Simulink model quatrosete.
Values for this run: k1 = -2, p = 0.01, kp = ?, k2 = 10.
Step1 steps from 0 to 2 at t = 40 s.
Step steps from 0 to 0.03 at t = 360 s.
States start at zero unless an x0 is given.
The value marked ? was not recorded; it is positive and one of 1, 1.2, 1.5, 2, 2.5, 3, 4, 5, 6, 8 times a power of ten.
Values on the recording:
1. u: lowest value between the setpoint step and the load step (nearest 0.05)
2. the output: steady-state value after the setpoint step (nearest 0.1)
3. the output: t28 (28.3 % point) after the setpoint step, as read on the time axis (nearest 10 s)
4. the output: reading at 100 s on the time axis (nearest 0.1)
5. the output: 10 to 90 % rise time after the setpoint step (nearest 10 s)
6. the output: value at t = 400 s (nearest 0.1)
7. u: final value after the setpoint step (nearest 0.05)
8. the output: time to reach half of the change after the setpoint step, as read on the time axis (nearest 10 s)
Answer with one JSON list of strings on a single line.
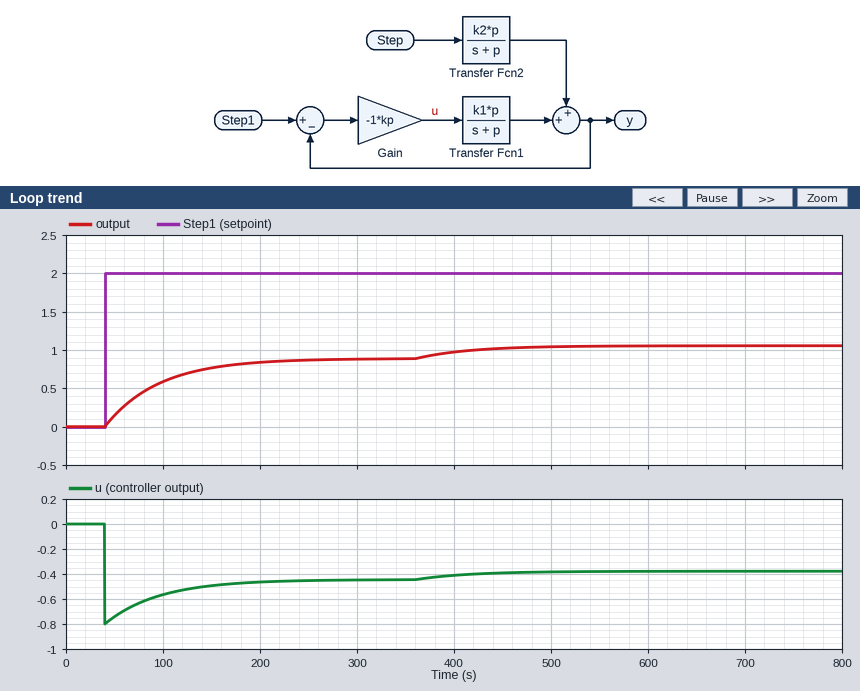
["-0.80", "0.9", "60 s", "0.6", "120 s", "1.0", "-0.45", "80 s"]
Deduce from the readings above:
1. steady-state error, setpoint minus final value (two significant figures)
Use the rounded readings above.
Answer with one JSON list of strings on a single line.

["1.1"]
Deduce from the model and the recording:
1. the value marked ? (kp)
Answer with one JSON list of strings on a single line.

["0.4"]
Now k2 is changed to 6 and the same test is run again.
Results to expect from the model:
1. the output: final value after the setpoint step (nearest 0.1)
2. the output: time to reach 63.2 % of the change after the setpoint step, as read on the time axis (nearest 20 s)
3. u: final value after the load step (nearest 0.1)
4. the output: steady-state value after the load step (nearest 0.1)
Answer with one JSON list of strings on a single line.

["0.9", "100 s", "-0.4", "1.0"]
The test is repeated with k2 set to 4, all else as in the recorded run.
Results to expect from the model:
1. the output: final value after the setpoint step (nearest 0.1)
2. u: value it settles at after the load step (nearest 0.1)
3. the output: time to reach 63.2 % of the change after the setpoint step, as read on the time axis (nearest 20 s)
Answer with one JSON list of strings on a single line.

["0.9", "-0.4", "100 s"]
